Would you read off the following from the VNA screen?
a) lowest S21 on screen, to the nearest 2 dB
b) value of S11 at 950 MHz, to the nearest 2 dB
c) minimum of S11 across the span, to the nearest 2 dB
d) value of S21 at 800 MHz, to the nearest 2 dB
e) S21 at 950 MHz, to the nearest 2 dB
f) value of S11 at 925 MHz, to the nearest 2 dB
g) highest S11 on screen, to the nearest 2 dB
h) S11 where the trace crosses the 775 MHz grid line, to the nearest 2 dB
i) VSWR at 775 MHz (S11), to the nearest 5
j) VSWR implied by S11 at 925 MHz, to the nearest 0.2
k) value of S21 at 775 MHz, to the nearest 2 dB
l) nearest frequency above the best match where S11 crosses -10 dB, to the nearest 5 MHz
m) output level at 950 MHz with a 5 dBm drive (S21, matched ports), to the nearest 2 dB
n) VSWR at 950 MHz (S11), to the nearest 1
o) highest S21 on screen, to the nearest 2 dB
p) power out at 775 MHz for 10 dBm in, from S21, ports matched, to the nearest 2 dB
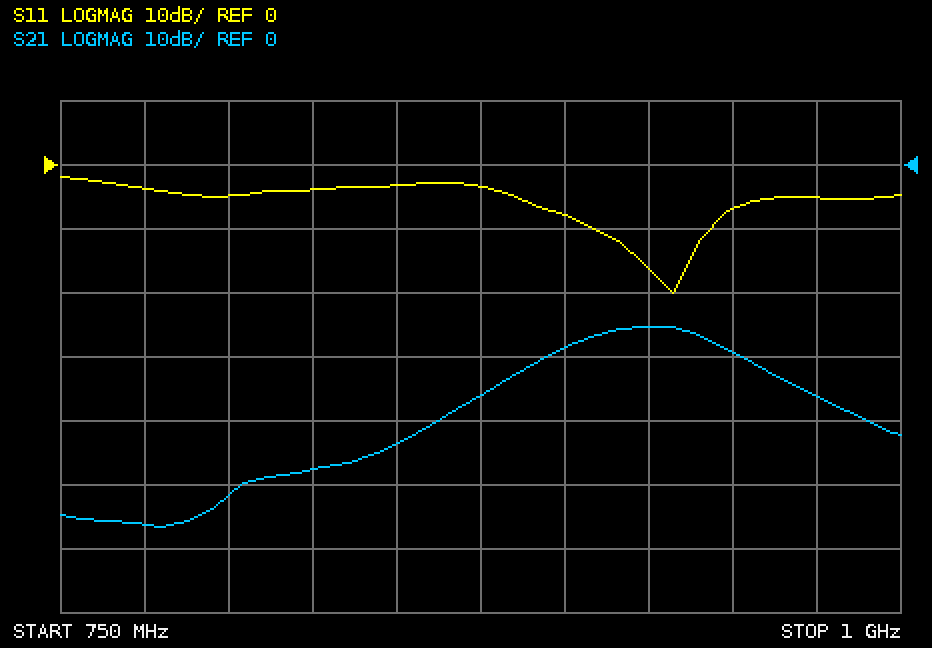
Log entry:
-56 dB
-6 dB
-20 dB
-52 dB
-30 dB
-16 dB
-2 dB
-4 dB
5
1.4
-56 dB
945 MHz
-24 dBm
3
-26 dB
-46 dBm
